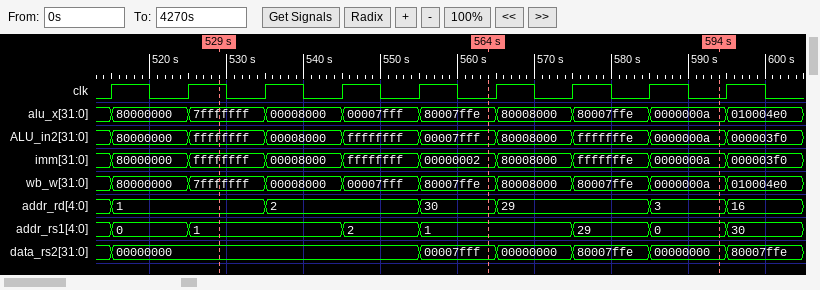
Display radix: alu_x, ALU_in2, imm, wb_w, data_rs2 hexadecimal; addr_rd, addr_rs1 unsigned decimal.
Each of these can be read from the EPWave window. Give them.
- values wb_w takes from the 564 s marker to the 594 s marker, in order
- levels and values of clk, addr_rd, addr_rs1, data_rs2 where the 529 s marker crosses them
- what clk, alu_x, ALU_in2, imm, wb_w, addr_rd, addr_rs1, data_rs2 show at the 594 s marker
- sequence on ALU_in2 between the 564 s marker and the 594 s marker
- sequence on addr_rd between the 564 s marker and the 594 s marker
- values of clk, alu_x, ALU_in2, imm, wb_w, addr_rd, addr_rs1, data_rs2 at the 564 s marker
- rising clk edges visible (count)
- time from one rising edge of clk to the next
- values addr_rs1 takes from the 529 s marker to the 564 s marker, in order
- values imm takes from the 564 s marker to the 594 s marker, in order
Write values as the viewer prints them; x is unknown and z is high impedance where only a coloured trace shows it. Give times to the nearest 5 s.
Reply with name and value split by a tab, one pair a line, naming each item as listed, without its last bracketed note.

values wb_w takes from the 564 s marker to the 594 s marker, in order	80007ffe, 80008000, 80007ffe, 0000000a
levels and values of clk, addr_rd, addr_rs1, data_rs2 where the 529 s marker crosses them	clk=1, addr_rd=1, addr_rs1=1, data_rs2=00000000
what clk, alu_x, ALU_in2, imm, wb_w, addr_rd, addr_rs1, data_rs2 show at the 594 s marker	clk=0, alu_x=0000000a, ALU_in2=0000000a, imm=0000000a, wb_w=0000000a, addr_rd=3, addr_rs1=0, data_rs2=00000000
sequence on ALU_in2 between the 564 s marker and the 594 s marker	00007fff, 80008000, fffffffe, 0000000a
sequence on addr_rd between the 564 s marker and the 594 s marker	30, 29, 3
values of clk, alu_x, ALU_in2, imm, wb_w, addr_rd, addr_rs1, data_rs2 at the 564 s marker	clk=0, alu_x=80007ffe, ALU_in2=00007fff, imm=00000002, wb_w=80007ffe, addr_rd=30, addr_rs1=1, data_rs2=00007fff
rising clk edges visible	9
time from one rising edge of clk to the next	10 s
values addr_rs1 takes from the 529 s marker to the 564 s marker, in order	1, 2, 1
values imm takes from the 564 s marker to the 594 s marker, in order	00000002, 80008000, fffffffe, 0000000a
